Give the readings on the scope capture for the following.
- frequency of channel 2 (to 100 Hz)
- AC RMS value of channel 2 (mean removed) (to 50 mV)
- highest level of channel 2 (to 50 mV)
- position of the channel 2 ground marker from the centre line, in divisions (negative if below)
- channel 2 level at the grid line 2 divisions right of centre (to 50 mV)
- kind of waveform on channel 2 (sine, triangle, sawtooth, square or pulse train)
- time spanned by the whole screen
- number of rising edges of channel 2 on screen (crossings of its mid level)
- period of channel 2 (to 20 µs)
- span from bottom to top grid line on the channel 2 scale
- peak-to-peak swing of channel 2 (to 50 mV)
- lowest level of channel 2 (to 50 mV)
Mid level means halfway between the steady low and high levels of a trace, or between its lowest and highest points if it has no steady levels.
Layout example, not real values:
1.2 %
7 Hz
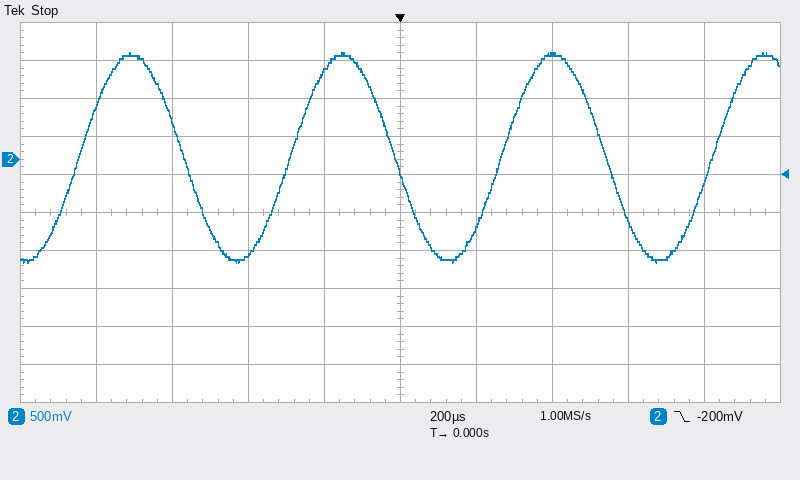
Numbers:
1.8 kHz
950 mV
1.40 V
+1.4 div
1.40 V
sine
2 ms
4
560 µs
5 V
2.75 V
-1.35 V
